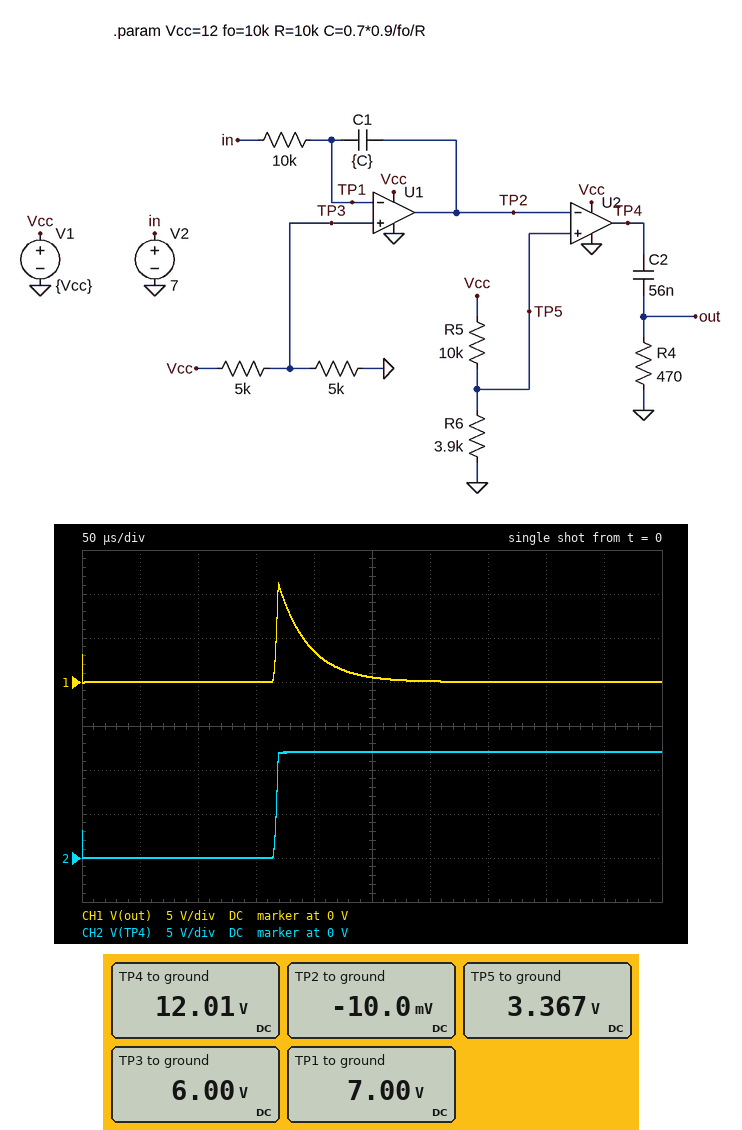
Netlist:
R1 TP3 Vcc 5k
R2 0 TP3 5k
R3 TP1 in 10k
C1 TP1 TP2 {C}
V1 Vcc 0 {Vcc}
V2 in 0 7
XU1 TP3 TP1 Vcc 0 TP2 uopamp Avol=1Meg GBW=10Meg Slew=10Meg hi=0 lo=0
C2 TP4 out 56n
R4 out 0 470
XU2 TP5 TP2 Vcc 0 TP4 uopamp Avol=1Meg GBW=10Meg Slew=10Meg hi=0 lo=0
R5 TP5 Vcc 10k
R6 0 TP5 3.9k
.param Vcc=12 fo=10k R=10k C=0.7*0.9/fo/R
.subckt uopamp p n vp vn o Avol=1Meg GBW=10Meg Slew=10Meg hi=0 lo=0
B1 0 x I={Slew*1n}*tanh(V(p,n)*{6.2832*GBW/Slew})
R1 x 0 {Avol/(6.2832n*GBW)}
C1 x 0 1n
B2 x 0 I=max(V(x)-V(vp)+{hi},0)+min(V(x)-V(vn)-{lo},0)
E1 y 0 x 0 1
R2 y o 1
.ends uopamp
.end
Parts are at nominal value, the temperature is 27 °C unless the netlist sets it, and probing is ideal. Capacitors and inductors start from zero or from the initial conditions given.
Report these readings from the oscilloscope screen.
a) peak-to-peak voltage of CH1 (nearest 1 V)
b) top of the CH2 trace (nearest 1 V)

11 V
12 V
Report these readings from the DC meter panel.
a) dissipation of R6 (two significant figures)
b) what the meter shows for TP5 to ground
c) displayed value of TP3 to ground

2.9 mW
3.367 V
6.00 V
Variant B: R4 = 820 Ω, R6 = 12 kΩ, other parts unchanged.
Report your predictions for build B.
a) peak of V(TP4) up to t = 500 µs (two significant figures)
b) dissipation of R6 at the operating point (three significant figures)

12 V
3.57 mW
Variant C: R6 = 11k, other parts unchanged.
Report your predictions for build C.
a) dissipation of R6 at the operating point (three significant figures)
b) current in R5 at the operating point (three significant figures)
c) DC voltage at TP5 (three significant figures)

3.59 mW
571 µA
6.29 V
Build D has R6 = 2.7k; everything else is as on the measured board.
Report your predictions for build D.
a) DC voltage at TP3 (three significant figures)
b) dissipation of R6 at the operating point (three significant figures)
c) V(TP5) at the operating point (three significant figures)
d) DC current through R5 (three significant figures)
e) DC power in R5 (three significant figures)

6.00 V
2.41 mW
2.55 V
945 µA
8.93 mW
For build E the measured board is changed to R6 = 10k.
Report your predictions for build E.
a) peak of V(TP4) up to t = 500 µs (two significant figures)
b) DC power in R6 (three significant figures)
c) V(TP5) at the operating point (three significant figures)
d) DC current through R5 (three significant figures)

12 V
3.60 mW
6.00 V
600 µA
